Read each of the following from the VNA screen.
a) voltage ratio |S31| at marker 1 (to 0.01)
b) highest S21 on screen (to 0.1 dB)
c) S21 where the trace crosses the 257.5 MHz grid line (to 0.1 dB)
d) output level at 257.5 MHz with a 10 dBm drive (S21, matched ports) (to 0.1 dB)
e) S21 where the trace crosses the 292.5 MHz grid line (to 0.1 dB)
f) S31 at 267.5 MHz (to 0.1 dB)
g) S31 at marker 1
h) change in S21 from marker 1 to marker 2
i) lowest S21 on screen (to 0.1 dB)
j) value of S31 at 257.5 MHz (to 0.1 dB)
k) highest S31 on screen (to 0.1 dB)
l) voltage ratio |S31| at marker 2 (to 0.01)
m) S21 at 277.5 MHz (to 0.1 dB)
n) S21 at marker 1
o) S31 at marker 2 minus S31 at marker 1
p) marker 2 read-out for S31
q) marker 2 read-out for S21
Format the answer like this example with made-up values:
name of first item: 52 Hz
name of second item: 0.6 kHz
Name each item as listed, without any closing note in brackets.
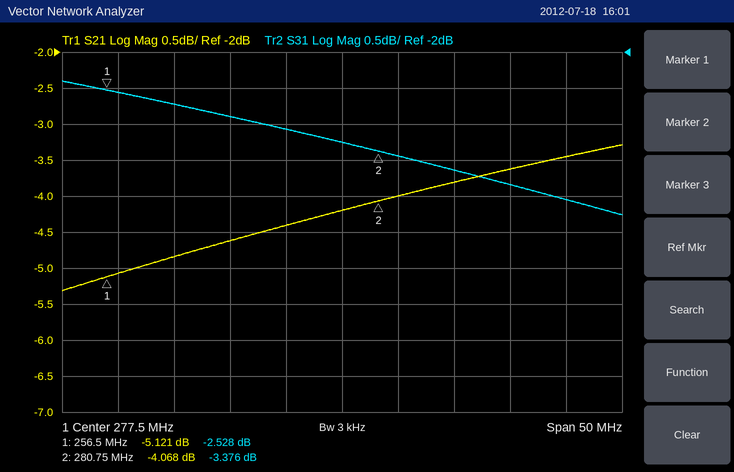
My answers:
voltage ratio |S31| at marker 1: 0.75
highest S21 on screen: -3.3 dB
S21 where the trace crosses the 257.5 MHz grid line: -5.1 dB
output level at 257.5 MHz with a 10 dBm drive (S21, matched ports): 4.9 dBm
S21 where the trace crosses the 292.5 MHz grid line: -3.6 dB
S31 at 267.5 MHz: -2.9 dB
S31 at marker 1: -2.528 dB
change in S21 from marker 1 to marker 2: 1.053 dB
lowest S21 on screen: -5.3 dB
value of S31 at 257.5 MHz: -2.6 dB
highest S31 on screen: -2.4 dB
voltage ratio |S31| at marker 2: 0.68
S21 at 277.5 MHz: -4.2 dB
S21 at marker 1: -5.121 dB
S31 at marker 2 minus S31 at marker 1: -0.848 dB
marker 2 read-out for S31: -3.376 dB
marker 2 read-out for S21: -4.068 dB
